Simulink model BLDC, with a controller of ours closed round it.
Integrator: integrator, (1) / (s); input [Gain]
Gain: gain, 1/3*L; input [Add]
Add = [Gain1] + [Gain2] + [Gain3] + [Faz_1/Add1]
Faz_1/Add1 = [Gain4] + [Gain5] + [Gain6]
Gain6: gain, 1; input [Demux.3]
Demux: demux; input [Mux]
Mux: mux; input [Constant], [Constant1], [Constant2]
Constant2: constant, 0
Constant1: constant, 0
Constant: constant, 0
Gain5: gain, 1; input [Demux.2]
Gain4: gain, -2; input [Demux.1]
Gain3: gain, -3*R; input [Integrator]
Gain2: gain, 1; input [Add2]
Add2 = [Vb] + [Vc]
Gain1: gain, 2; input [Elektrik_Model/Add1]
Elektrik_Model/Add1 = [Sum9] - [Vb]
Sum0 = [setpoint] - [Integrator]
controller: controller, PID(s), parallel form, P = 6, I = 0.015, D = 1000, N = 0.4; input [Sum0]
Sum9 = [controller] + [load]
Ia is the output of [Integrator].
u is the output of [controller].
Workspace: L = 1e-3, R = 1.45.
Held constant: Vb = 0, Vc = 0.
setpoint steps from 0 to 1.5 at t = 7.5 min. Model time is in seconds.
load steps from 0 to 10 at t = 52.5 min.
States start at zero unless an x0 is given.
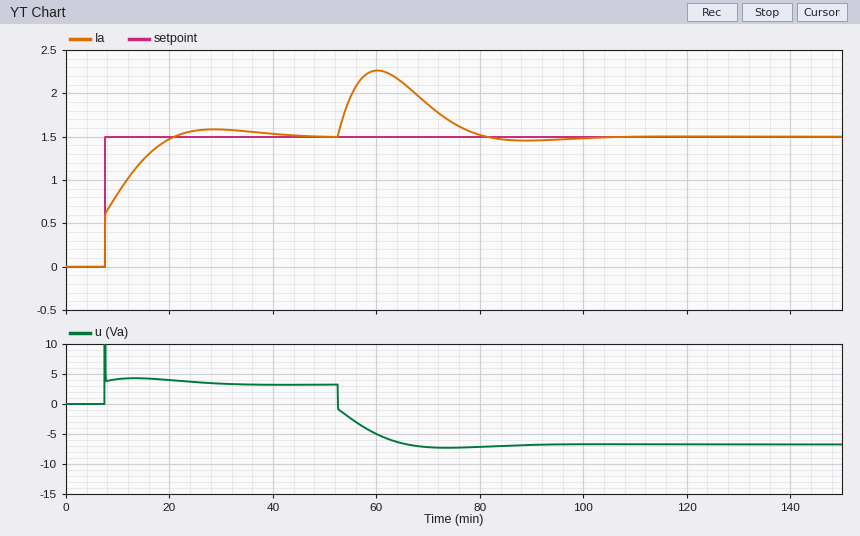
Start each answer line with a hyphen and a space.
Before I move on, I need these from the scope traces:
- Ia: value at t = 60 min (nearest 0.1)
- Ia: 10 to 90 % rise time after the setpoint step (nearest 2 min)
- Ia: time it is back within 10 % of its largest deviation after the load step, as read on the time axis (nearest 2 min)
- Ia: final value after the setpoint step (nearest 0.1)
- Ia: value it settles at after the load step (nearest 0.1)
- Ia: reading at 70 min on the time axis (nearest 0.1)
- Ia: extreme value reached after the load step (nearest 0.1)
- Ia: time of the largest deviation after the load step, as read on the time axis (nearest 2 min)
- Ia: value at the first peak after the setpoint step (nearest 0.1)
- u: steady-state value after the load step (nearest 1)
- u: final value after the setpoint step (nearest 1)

- 2.3
- 10 min
- 78 min
- 1.5
- 1.5
- 1.9
- 2.3
- 60 min
- 1.6
- -7
- 3
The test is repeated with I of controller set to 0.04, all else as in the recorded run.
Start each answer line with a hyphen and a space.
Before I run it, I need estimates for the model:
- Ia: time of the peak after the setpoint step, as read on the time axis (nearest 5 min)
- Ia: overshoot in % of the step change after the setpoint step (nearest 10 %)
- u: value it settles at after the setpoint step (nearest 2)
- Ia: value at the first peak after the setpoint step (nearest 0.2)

- 20 min
- 20 %
- 4
- 1.8
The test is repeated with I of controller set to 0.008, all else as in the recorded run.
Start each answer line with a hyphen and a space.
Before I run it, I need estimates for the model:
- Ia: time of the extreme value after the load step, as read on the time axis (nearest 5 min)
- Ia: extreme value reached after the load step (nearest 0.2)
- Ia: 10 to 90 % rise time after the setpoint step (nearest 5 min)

- 60 min
- 2.4
- 15 min
